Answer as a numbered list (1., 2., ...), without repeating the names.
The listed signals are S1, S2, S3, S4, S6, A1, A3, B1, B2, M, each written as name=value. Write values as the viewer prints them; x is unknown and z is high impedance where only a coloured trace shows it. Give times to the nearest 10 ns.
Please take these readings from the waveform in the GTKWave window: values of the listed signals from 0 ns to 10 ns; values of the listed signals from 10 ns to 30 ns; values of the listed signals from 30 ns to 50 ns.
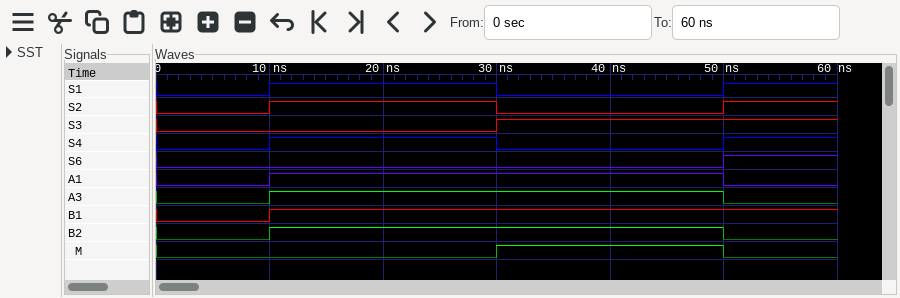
1. S1=0, S2=0, S3=0, S4=0, S6=0, A1=0, A3=0, B1=0, B2=0, M=0
2. S1=1, S2=1, S3=0, S4=1, S6=0, A1=1, A3=1, B1=1, B2=1, M=0
3. S1=0, S2=0, S3=1, S4=0, S6=0, A1=1, A3=1, B1=1, B2=1, M=1
